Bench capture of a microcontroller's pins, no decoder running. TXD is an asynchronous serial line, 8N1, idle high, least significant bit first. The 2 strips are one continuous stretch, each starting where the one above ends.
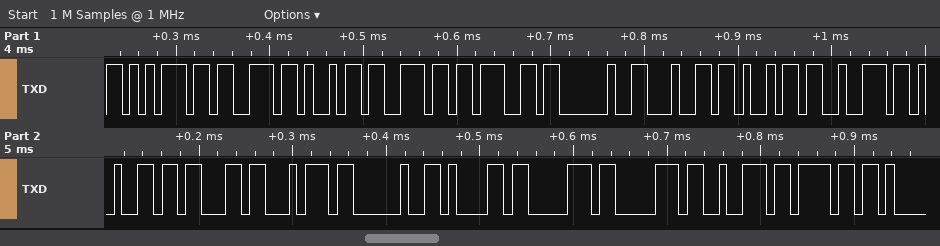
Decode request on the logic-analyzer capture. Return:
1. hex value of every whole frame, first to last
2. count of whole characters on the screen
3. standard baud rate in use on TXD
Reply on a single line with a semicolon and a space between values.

75 73 69 6E 67 20 64 69 72 65 63 74 20 61 70 70 72 6F; 18; 115200 baud
